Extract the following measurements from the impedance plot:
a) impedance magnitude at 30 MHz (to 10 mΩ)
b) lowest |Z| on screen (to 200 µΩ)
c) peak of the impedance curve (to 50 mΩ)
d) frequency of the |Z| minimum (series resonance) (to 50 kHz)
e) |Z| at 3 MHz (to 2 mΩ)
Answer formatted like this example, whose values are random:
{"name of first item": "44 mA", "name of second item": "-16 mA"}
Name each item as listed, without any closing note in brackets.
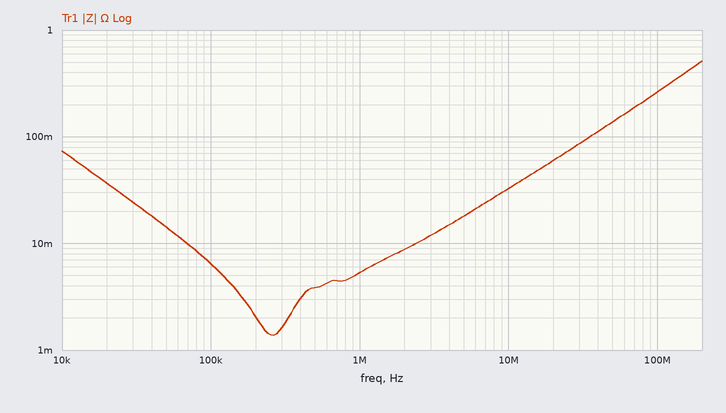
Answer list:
{"impedance magnitude at 30 MHz": "90 mΩ", "lowest |Z| on screen": "1.4 mΩ", "peak of the impedance curve": "500 mΩ", "frequency of the |Z| minimum (series resonance)": "250 kHz", "|Z| at 3 MHz": "12 mΩ"}
